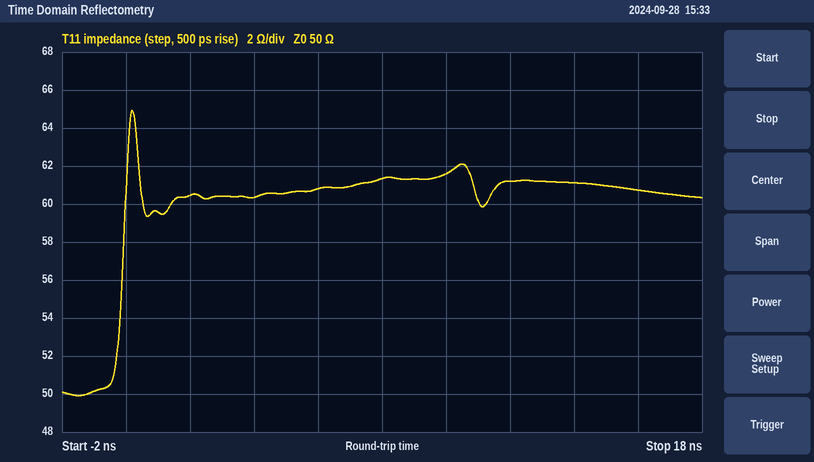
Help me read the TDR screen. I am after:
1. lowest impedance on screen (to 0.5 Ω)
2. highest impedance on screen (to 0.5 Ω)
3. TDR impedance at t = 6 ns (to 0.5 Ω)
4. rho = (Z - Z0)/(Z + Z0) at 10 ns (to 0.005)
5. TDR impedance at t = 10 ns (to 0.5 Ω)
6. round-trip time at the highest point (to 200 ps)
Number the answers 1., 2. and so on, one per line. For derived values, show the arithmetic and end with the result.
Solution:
1. 50.0 Ω
2. 65.0 Ω
3. 61.0 Ω
4. (61.5 − 50)/(61.5 + 50) ≈ +0.103, so +0.105 to the nearest 0.005
5. 61.5 Ω
6. 200 ps
